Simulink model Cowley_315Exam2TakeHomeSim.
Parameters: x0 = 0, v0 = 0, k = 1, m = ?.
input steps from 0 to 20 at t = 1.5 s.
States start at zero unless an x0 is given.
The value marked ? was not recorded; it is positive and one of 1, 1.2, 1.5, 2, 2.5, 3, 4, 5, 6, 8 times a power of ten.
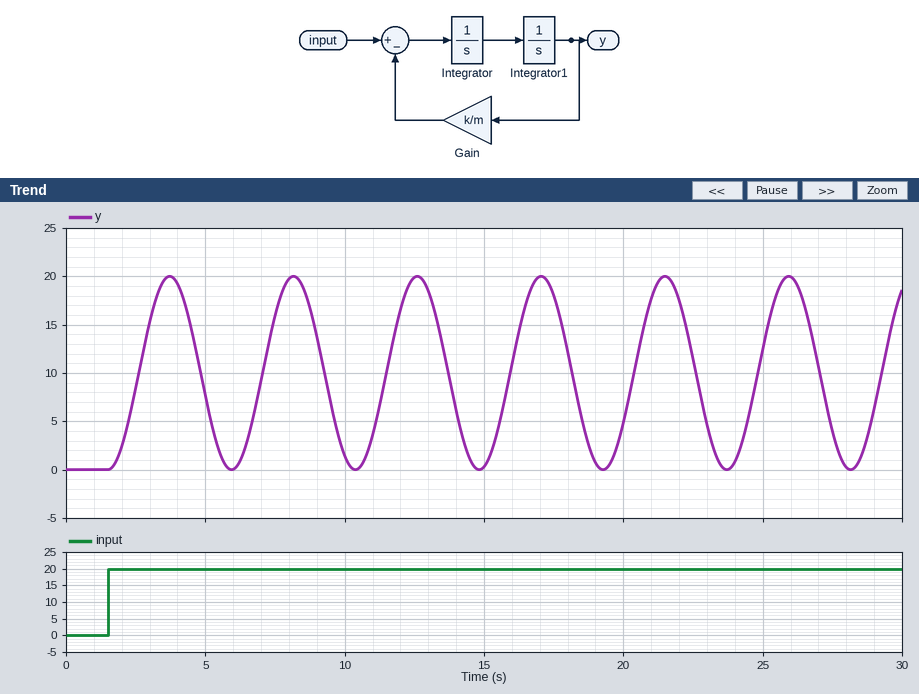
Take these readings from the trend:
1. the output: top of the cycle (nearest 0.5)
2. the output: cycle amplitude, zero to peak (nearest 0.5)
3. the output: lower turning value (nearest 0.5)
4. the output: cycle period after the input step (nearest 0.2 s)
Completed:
20.0
10.0
0.0
4.4 s
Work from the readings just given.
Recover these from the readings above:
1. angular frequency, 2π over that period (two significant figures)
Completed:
1.4 rad/s
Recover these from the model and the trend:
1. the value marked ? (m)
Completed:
0.5
